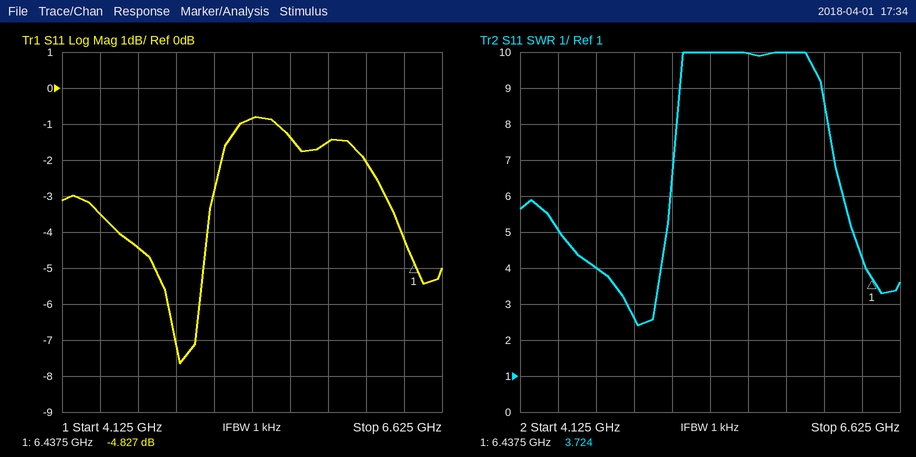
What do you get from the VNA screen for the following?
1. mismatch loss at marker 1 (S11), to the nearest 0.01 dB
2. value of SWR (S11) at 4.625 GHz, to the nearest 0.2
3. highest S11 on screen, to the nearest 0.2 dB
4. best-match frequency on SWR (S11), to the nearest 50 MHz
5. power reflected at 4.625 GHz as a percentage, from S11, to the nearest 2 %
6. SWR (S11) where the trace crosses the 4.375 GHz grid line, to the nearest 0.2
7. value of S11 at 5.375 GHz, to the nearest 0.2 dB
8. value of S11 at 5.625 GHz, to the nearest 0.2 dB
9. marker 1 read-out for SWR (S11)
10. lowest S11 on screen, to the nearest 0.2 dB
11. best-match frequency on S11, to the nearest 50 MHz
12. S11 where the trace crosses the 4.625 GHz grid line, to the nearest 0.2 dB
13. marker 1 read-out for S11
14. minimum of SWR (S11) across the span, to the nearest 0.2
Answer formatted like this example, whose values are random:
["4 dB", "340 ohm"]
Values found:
["1.73 dB", "4.0", "-0.8 dB", "4.90 GHz", "36 %", "5.0", "-0.8 dB", "-1.4 dB", "3.724", "-7.6 dB", "4.90 GHz", "-4.4 dB", "-4.827 dB", "2.4"]
